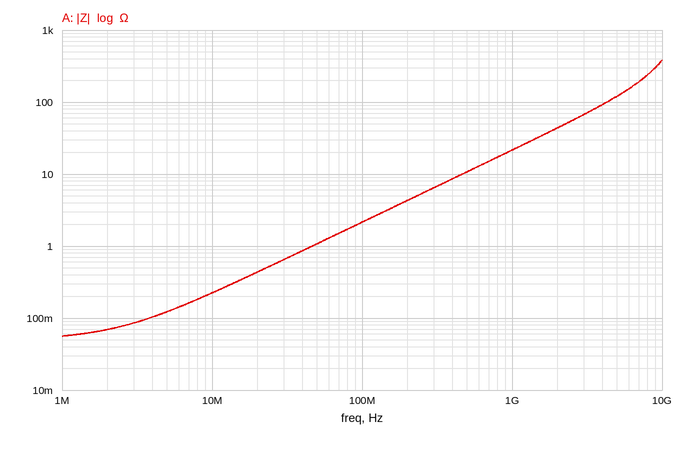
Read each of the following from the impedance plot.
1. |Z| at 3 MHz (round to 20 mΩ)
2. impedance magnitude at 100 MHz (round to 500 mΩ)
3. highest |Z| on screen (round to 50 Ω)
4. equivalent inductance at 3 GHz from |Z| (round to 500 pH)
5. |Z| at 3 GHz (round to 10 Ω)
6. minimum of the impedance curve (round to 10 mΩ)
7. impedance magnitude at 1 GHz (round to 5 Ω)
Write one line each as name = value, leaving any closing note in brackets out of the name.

|Z| at 3 MHz = 80 mΩ
impedance magnitude at 100 MHz = 2.0 Ω
highest |Z| on screen = 400 Ω
equivalent inductance at 3 GHz from |Z| = 3.5 nH
|Z| at 3 GHz = 70 Ω
minimum of the impedance curve = 60 mΩ
impedance magnitude at 1 GHz = 20 Ω
